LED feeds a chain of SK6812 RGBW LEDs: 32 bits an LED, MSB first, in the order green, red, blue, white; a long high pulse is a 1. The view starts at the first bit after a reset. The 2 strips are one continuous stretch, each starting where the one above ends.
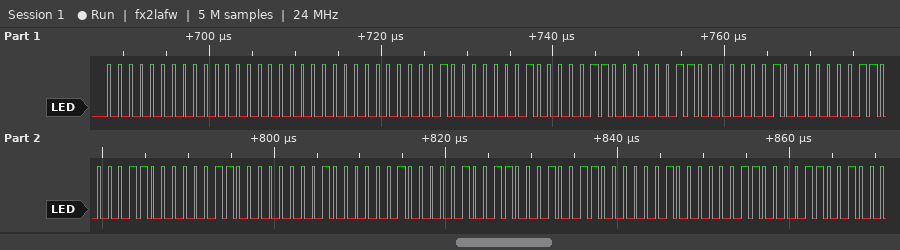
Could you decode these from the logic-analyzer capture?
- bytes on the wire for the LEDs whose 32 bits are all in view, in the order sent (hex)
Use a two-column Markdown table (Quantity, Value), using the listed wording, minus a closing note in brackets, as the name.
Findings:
| Quantity | Value |
|---|---|
| bytes on the wire for the LEDs whose 32 bits are all in view, in the order sent | 00 00 00 01 01 06 06 02 03 0C 0C 02 04 13 13 02 |
